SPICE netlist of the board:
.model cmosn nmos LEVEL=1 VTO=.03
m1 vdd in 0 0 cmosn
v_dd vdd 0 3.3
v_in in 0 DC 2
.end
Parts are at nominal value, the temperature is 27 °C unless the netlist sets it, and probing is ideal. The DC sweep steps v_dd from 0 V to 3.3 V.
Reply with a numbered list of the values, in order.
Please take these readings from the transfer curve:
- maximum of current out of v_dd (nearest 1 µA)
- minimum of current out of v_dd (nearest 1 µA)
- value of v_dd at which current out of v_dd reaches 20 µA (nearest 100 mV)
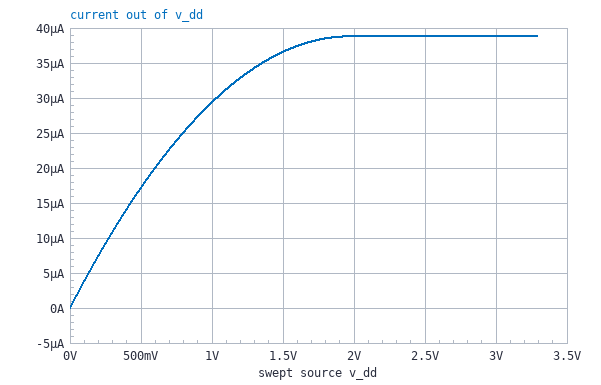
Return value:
1. 39 µA
2. 0 A
3. 600 mV
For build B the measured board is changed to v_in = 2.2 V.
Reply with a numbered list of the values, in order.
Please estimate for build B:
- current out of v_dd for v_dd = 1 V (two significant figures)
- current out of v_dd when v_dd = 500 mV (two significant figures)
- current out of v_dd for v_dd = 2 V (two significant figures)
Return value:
1. 33 µA
2. 19 µA
3. 47 µA
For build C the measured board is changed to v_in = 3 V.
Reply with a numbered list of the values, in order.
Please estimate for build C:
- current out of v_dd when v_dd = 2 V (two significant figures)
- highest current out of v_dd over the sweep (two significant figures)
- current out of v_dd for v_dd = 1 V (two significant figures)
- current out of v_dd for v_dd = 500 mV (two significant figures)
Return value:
1. 79 µA
2. 88 µA
3. 49 µA
4. 27 µA
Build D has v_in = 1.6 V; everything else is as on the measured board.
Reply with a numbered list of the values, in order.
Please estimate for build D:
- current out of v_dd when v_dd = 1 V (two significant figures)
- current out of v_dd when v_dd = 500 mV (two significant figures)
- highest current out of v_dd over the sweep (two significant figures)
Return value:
1. 21 µA
2. 13 µA
3. 25 µA
